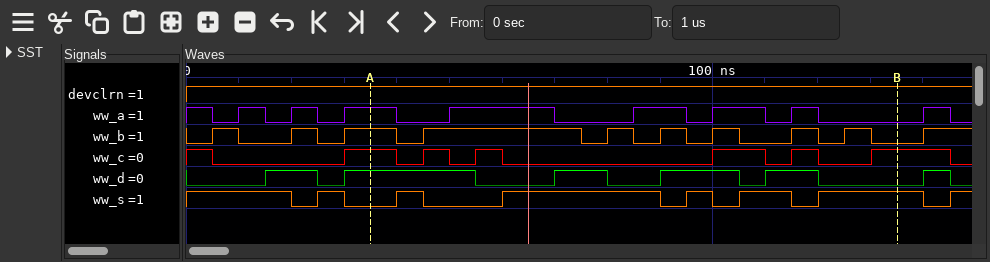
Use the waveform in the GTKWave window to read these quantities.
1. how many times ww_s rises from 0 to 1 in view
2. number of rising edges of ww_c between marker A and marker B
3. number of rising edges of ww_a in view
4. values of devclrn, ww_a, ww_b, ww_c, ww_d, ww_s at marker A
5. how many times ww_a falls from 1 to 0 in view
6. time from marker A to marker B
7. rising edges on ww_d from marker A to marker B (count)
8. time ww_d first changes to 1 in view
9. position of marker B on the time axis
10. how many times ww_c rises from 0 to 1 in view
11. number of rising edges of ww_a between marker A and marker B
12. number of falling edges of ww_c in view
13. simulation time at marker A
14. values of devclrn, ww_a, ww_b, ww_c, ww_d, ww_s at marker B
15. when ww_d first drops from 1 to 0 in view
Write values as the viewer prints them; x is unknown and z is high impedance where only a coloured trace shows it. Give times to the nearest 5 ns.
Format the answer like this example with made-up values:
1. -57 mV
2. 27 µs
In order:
1. 7
2. 5
3. 8
4. devclrn=1, ww_a=1, ww_b=1, ww_c=1, ww_d=1, ww_s=0
5. 9
6. 100 ns
7. 3
8. 15 ns
9. 135 ns
10. 6
11. 4
12. 7
13. 35 ns
14. devclrn=1, ww_a=0, ww_b=0, ww_c=1, ww_d=0, ww_s=1
15. 25 ns
